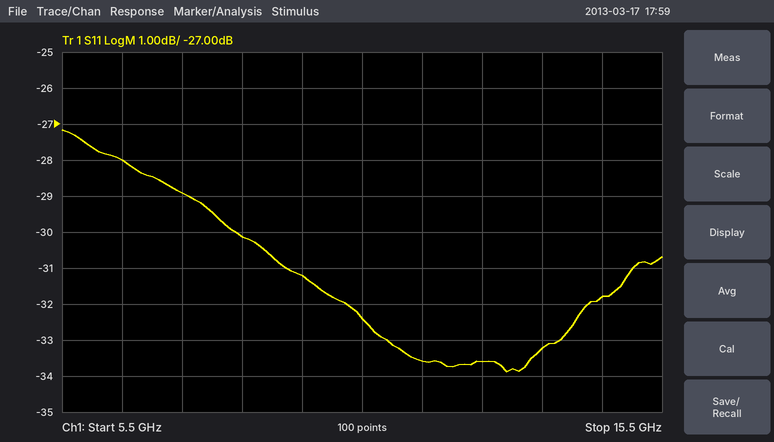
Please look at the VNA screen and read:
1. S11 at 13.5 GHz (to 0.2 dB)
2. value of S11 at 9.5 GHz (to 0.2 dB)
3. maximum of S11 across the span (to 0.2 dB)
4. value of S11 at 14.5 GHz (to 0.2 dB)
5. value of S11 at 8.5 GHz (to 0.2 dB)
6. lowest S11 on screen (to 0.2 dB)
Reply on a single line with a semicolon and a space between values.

-33.2 dB; -31.2 dB; -27.2 dB; -31.8 dB; -30.2 dB; -33.8 dB
